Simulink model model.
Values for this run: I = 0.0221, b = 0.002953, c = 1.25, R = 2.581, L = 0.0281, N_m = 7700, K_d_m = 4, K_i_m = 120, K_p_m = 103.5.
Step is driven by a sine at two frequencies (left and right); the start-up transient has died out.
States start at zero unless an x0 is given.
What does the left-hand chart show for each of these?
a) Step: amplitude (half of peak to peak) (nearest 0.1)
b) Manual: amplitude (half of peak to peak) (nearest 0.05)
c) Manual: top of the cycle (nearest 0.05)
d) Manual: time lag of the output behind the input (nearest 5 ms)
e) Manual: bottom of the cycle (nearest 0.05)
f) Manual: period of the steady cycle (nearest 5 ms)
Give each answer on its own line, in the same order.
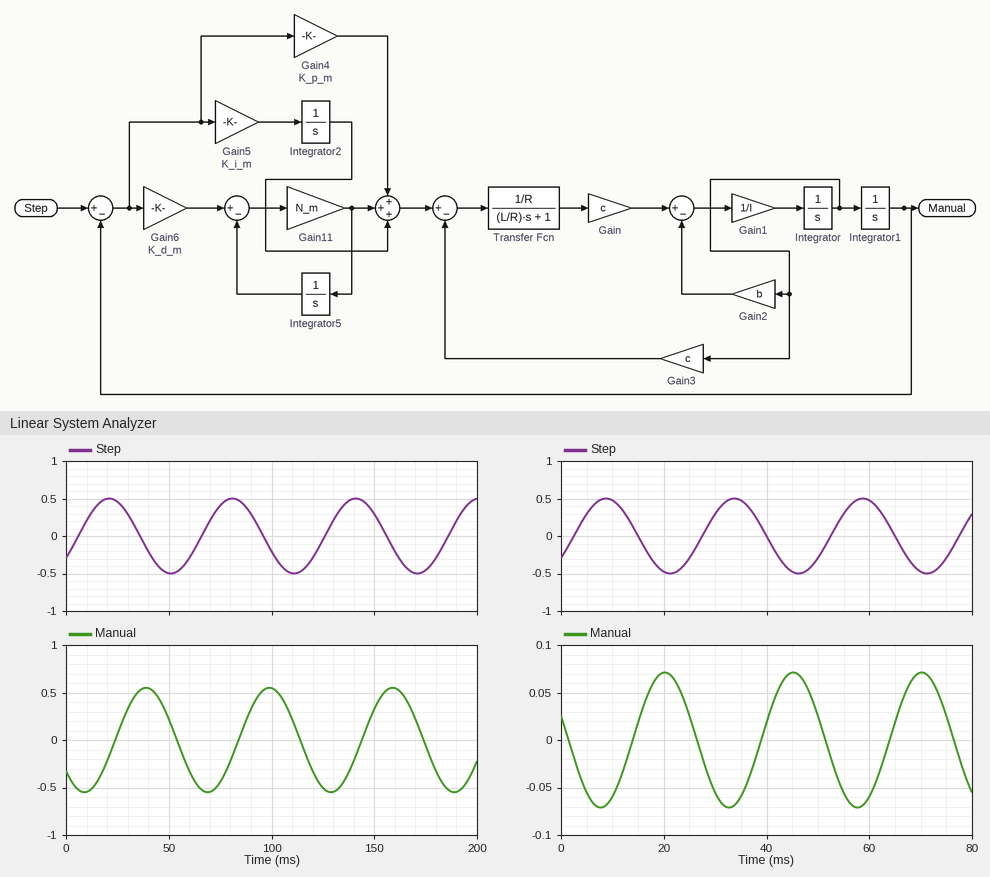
0.5
0.55
0.55
20 ms
-0.55
60 ms
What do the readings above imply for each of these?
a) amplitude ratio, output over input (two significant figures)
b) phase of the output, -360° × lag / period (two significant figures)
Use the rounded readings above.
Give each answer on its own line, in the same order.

1.1
-120°
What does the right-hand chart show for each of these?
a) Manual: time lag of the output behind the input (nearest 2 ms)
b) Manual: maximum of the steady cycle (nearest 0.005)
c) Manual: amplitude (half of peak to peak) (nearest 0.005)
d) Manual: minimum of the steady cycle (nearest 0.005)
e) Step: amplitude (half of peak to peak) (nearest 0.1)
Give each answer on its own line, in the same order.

12 ms
0.070
0.070
-0.070
0.5
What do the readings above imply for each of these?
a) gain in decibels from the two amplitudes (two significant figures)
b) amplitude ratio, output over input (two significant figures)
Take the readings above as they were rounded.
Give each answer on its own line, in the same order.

-17 dB
0.14
